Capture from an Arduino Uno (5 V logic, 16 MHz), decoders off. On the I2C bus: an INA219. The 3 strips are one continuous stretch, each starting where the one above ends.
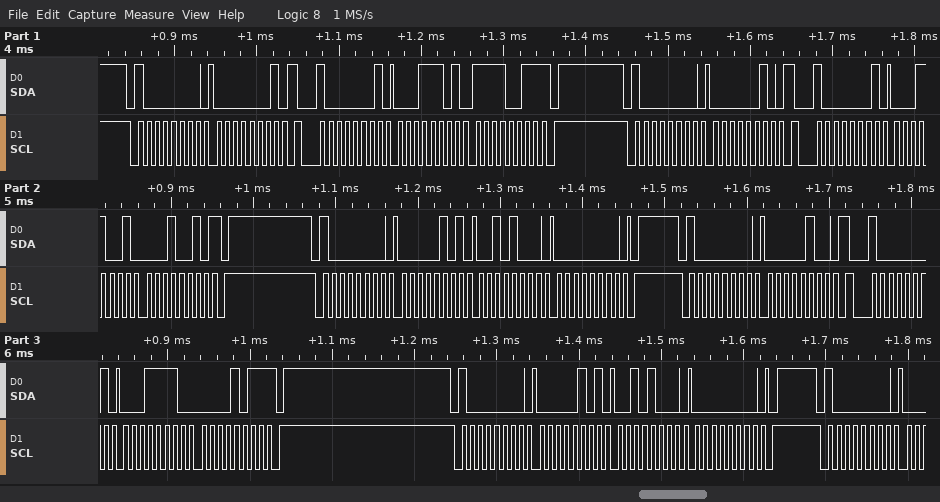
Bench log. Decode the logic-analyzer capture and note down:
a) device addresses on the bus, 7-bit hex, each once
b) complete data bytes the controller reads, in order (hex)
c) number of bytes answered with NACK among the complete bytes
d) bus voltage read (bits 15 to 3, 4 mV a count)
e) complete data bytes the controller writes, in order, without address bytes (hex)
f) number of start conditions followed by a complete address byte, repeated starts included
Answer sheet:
0x40
1D F3 19 12 1E 0B
3
3.208 V
01 02 05 28 00 04 05 28 00
9
